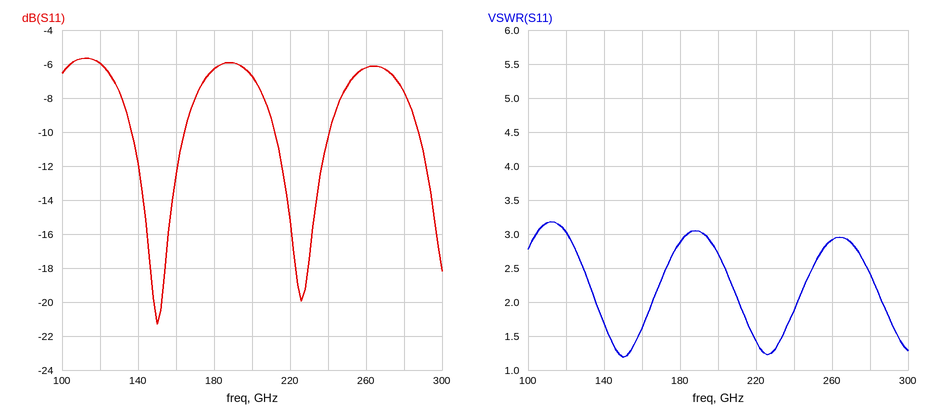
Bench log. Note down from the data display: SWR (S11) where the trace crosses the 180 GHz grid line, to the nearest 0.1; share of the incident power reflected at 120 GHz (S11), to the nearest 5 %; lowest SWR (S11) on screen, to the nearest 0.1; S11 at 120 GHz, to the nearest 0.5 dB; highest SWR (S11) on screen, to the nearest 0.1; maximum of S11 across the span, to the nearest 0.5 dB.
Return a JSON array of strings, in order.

["2.9", "25 %", "1.2", "-6.0 dB", "3.2", "-5.5 dB"]
